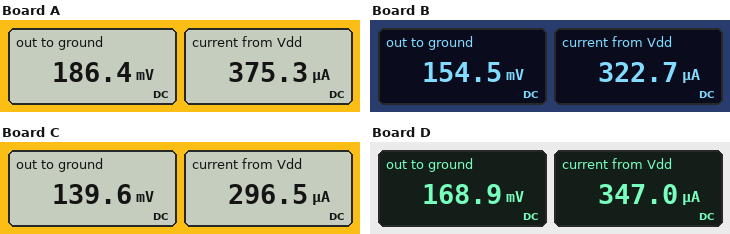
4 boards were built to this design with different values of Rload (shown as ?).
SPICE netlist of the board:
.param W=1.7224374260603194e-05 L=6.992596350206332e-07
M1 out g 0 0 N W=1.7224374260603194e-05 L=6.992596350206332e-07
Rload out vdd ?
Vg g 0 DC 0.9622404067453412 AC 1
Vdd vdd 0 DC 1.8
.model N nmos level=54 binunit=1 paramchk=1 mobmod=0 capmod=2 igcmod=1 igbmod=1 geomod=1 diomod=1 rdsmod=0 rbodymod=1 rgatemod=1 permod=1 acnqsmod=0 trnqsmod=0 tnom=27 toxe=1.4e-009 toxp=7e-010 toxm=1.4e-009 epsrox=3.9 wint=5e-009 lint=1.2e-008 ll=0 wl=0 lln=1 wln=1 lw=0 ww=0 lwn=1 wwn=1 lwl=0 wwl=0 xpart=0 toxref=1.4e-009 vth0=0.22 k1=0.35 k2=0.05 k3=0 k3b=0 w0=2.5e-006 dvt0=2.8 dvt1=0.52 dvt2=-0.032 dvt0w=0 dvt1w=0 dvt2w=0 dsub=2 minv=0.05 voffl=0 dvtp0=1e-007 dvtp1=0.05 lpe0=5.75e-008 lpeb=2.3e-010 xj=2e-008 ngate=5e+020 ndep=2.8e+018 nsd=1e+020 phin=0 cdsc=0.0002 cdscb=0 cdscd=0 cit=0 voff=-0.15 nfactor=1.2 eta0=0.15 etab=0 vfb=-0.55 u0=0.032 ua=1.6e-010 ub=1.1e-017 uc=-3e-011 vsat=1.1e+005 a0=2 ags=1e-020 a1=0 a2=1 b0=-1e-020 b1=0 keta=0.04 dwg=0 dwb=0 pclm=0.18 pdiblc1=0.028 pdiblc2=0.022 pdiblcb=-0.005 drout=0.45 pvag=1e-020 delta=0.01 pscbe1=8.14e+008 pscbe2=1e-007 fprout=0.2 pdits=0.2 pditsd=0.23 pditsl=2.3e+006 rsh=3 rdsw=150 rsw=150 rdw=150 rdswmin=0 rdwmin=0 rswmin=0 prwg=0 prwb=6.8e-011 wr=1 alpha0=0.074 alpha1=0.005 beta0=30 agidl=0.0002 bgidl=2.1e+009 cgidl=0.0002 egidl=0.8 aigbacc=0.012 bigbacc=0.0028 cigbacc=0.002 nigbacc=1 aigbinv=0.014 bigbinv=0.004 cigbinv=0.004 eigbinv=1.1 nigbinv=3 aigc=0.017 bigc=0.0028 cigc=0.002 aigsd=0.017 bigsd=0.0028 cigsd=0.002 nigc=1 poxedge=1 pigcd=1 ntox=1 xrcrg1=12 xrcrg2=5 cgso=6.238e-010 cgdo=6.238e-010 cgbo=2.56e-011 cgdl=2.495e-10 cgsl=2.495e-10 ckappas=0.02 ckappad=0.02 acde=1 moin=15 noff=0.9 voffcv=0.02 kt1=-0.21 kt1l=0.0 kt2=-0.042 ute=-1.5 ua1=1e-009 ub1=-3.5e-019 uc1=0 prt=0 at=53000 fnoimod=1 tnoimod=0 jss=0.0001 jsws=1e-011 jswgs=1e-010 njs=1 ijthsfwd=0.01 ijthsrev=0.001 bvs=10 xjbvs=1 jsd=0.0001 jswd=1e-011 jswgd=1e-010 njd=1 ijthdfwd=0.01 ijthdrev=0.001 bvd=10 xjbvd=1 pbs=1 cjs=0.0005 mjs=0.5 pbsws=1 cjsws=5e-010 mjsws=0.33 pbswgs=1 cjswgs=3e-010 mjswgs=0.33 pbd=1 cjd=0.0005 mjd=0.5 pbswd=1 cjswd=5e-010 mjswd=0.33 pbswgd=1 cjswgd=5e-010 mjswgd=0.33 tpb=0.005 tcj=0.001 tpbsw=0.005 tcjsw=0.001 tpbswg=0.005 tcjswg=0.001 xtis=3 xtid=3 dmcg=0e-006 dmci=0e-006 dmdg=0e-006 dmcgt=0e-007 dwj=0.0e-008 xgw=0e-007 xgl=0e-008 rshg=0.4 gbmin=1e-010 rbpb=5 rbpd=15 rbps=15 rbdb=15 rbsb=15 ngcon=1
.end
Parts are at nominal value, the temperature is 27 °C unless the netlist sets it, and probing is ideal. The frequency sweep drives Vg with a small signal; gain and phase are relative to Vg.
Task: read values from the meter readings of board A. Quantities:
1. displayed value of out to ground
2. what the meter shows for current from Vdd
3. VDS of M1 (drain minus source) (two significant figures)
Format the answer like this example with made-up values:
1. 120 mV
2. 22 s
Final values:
1. 186.4 mV
2. 375.3 µA
3. 190 mV
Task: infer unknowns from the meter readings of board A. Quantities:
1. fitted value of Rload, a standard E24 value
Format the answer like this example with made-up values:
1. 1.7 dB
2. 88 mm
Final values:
1. 4.3 kΩ
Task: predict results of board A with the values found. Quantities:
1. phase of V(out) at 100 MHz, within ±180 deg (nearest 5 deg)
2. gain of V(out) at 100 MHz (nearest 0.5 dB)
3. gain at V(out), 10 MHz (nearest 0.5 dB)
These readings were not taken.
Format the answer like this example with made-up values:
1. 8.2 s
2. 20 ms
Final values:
1. 130 deg
2. -19.5 dB
3. -22.5 dB
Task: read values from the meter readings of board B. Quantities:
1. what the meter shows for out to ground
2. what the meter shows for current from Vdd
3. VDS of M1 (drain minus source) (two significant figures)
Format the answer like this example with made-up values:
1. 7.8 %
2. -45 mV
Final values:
1. 154.5 mV
2. 322.7 µA
3. 150 mV
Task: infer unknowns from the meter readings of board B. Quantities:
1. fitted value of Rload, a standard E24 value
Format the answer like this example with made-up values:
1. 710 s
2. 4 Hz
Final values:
1. 5.1 kΩ
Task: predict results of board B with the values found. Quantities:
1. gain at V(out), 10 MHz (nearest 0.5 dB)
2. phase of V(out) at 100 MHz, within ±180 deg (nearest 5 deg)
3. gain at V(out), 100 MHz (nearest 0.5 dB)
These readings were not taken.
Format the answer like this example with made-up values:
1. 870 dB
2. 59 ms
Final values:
1. -25.5 dB
2. 120 deg
3. -21.0 dB
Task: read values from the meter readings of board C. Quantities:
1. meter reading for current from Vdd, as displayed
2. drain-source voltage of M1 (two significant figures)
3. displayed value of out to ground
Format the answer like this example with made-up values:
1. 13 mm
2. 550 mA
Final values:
1. 296.5 µA
2. 140 mV
3. 139.6 mV
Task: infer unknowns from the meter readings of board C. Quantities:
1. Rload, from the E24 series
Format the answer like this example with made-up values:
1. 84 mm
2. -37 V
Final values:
1. 5.6 kΩ
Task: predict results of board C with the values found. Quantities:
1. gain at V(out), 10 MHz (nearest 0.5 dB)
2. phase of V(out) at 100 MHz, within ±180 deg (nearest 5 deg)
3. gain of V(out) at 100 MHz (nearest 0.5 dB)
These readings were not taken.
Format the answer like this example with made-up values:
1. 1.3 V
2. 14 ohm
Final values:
1. -27.5 dB
2. 115 deg
3. -21.5 dB
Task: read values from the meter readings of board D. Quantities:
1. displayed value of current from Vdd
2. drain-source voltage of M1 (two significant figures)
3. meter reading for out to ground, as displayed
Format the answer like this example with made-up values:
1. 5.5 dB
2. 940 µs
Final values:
1. 347.0 µA
2. 170 mV
3. 168.9 mV
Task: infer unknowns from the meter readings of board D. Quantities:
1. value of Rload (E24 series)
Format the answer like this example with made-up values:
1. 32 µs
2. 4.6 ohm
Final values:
1. 4.7 kΩ
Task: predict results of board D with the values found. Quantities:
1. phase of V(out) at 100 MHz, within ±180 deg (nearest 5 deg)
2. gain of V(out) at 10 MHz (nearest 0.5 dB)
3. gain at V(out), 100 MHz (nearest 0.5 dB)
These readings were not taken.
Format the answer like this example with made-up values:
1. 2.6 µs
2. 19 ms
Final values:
1. 125 deg
2. -24.0 dB
3. -20.0 dB
